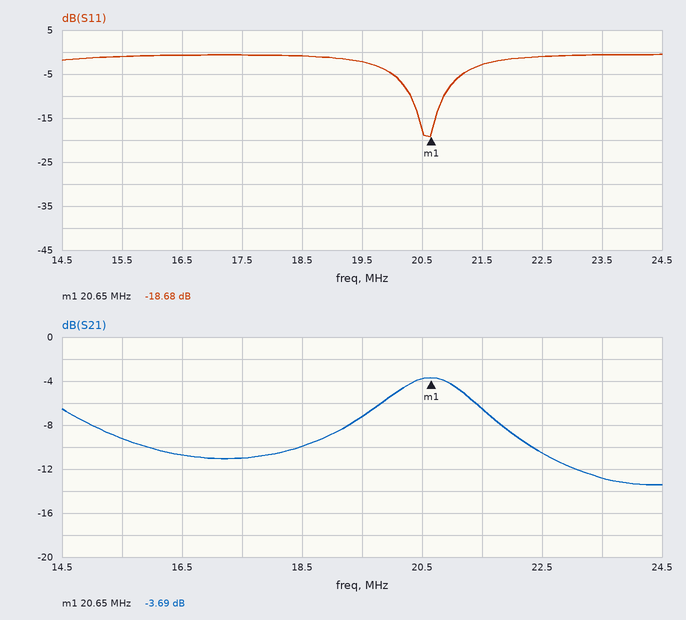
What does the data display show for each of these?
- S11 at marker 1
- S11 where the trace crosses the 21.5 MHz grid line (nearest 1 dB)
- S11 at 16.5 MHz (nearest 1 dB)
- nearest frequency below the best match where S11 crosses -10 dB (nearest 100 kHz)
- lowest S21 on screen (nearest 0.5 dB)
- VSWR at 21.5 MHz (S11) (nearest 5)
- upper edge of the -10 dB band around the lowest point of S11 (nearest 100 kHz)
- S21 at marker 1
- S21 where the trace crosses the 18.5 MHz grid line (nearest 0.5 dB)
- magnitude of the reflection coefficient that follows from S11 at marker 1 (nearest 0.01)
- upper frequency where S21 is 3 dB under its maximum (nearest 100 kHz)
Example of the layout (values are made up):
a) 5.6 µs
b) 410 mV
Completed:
a) -18.68 dB
b) -3 dB
c) -1 dB
d) 20.3 MHz
e) -13.5 dB
f) 5
g) 20.9 MHz
h) -3.69 dB
i) -10.0 dB
j) 0.12
k) 21.5 MHz
